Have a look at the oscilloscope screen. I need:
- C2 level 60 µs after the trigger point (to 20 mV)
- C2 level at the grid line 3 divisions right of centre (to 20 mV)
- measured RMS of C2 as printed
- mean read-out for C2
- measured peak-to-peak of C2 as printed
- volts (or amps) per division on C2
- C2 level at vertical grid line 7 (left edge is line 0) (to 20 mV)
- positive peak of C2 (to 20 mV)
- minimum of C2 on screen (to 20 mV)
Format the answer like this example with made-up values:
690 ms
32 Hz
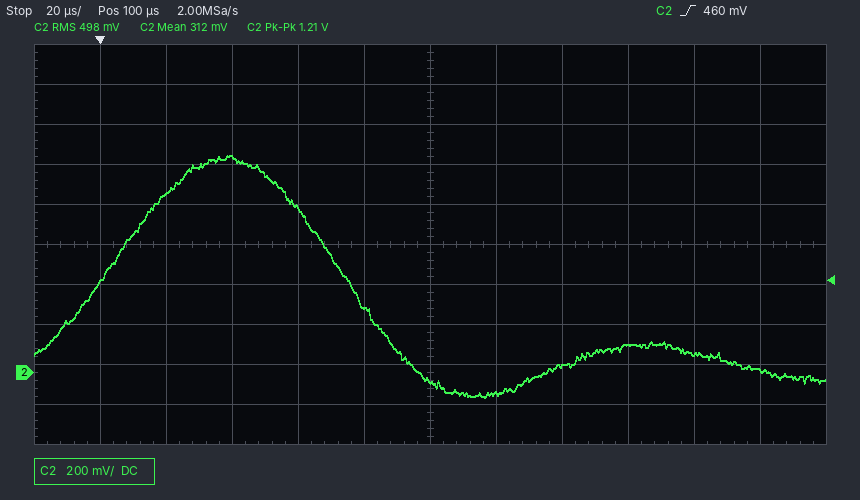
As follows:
820 mV
140 mV
498 mV
312 mV
1.21 V
200 mV
-100 mV
1.08 V
-120 mV
